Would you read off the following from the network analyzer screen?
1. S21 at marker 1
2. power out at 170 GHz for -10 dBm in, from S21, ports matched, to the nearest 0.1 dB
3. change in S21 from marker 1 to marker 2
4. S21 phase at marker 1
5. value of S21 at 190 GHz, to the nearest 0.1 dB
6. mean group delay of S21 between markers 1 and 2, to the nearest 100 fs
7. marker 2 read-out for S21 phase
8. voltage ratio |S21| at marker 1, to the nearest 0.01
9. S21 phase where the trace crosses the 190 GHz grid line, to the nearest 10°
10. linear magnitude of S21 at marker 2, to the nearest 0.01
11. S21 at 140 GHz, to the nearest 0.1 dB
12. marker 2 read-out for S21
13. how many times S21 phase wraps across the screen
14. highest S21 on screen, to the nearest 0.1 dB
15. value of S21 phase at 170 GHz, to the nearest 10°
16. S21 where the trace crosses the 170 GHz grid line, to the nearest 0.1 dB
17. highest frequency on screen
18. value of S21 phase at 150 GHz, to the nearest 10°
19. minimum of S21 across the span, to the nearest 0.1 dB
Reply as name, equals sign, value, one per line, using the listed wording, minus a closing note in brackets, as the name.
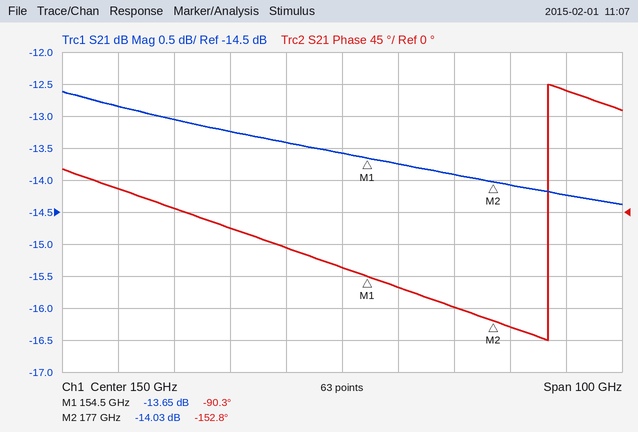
S21 at marker 1 = -13.65 dB
power out at 170 GHz for -10 dBm in, from S21, ports matched, to the nearest 0.1 dB = -23.9 dBm
change in S21 from marker 1 to marker 2 = -0.38 dB
S21 phase at marker 1 = -90.3°
value of S21 at 190 GHz, to the nearest 0.1 dB = -14.2 dB
mean group delay of S21 between markers 1 and 2, to the nearest 100 fs = 7.7 ps
marker 2 read-out for S21 phase = -152.8°
voltage ratio |S21| at marker 1, to the nearest 0.01 = 0.21
S21 phase where the trace crosses the 190 GHz grid line, to the nearest 10° = 170°
linear magnitude of S21 at marker 2, to the nearest 0.01 = 0.20
S21 at 140 GHz, to the nearest 0.1 dB = -13.4 dB
marker 2 read-out for S21 = -14.03 dB
how many times S21 phase wraps across the screen = 1
highest S21 on screen, to the nearest 0.1 dB = -12.6 dB
value of S21 phase at 170 GHz, to the nearest 10° = -130°
S21 where the trace crosses the 170 GHz grid line, to the nearest 0.1 dB = -13.9 dB
highest frequency on screen = 200 GHz
value of S21 phase at 150 GHz, to the nearest 10° = -80°
minimum of S21 across the span, to the nearest 0.1 dB = -14.4 dB
